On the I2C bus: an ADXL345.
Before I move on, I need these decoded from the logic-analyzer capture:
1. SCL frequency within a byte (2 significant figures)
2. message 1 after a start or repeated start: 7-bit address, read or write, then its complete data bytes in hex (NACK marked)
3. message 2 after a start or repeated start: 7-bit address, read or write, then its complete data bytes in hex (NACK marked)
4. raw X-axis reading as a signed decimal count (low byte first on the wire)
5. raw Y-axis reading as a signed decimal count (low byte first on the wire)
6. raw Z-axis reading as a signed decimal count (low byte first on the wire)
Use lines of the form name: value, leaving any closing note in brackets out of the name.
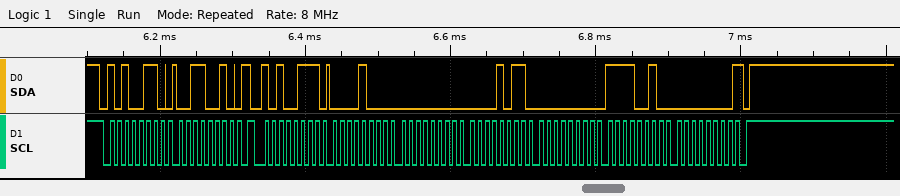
SCL frequency within a byte: 100 kHz
message 1 after a start or repeated start: 7-bit address, read or write, then its complete data bytes in hex: 0x53 write: 32
message 2 after a start or repeated start: 7-bit address, read or write, then its complete data bytes in hex: 0x53 read: 08 00 0B 00 F2 00 NACK
raw X-axis reading as a signed decimal count: 8
raw Y-axis reading as a signed decimal count: 11
raw Z-axis reading as a signed decimal count: 242
